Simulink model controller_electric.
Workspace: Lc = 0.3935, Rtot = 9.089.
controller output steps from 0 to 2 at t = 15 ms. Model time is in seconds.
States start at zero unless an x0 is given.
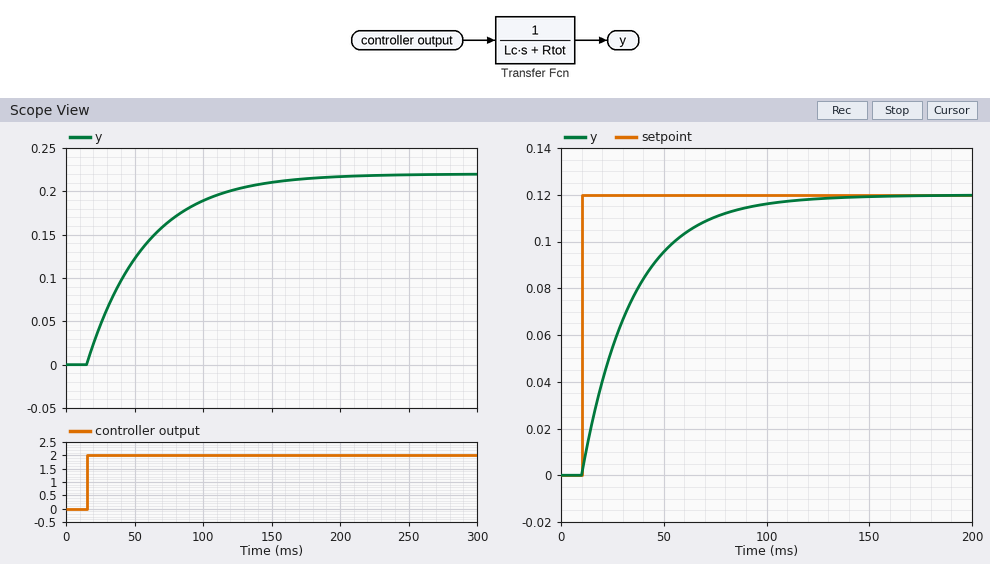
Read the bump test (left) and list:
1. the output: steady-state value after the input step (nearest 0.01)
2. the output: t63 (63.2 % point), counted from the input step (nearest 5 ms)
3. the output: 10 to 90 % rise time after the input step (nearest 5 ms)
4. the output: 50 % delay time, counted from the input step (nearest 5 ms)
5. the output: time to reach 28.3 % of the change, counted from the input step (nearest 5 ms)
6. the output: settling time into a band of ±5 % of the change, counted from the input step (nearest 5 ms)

0.22
45 ms
95 ms
30 ms
15 ms
130 ms
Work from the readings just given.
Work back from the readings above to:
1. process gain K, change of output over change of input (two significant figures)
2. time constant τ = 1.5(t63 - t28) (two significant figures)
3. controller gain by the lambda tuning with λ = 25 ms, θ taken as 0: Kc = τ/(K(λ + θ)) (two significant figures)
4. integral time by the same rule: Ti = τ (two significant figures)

0.11
45 ms
16
45 ms
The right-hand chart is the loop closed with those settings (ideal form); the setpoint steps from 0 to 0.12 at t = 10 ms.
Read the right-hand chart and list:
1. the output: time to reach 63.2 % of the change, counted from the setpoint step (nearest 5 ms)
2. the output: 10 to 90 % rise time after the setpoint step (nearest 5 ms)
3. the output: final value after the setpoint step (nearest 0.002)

25 ms
55 ms
0.120
